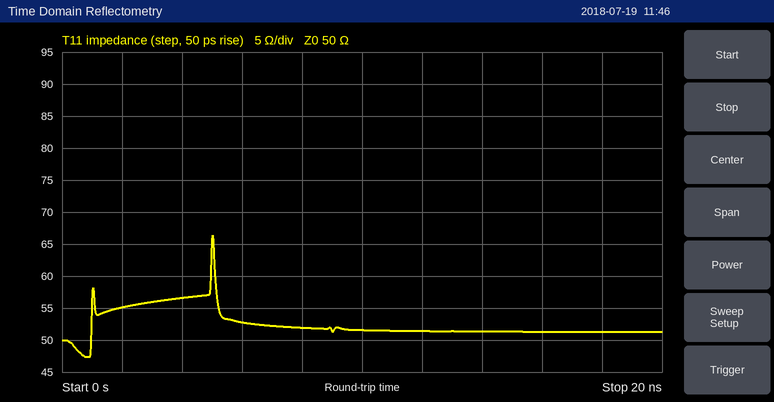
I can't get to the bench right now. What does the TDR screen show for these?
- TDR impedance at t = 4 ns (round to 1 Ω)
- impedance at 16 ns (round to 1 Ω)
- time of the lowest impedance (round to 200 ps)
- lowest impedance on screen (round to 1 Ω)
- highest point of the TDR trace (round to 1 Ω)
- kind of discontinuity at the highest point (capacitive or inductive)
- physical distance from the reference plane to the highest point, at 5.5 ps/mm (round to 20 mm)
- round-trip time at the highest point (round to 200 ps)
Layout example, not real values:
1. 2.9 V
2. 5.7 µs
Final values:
1. 57 Ω
2. 51 Ω
3. 800 ps
4. 47 Ω
5. 66 Ω
6. inductive
7. 460 mm
8. 5.0 ns
